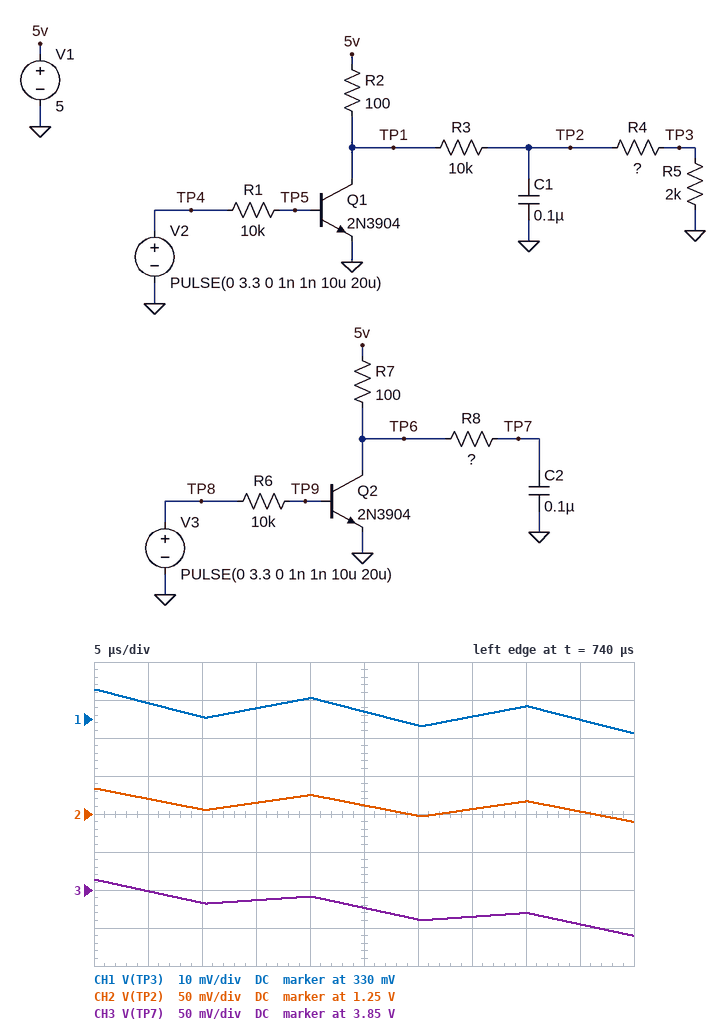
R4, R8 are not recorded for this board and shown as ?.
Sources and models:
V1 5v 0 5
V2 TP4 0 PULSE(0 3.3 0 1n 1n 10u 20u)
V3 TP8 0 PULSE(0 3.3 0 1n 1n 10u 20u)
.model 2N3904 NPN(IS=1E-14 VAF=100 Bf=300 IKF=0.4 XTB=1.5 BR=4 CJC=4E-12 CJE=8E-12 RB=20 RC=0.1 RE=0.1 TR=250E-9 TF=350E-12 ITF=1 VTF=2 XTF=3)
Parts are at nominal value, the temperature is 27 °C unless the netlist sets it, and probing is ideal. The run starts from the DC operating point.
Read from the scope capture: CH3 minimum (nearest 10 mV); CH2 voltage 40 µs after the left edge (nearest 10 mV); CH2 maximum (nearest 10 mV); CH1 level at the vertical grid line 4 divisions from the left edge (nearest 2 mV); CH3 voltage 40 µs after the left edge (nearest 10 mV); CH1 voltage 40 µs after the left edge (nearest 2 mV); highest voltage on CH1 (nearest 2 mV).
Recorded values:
3.79 V
1.27 V
1.28 V
336 mV
3.82 V
334 mV
338 mV
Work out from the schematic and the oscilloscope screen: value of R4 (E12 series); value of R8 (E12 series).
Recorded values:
5.6 kΩ
12 kΩ
